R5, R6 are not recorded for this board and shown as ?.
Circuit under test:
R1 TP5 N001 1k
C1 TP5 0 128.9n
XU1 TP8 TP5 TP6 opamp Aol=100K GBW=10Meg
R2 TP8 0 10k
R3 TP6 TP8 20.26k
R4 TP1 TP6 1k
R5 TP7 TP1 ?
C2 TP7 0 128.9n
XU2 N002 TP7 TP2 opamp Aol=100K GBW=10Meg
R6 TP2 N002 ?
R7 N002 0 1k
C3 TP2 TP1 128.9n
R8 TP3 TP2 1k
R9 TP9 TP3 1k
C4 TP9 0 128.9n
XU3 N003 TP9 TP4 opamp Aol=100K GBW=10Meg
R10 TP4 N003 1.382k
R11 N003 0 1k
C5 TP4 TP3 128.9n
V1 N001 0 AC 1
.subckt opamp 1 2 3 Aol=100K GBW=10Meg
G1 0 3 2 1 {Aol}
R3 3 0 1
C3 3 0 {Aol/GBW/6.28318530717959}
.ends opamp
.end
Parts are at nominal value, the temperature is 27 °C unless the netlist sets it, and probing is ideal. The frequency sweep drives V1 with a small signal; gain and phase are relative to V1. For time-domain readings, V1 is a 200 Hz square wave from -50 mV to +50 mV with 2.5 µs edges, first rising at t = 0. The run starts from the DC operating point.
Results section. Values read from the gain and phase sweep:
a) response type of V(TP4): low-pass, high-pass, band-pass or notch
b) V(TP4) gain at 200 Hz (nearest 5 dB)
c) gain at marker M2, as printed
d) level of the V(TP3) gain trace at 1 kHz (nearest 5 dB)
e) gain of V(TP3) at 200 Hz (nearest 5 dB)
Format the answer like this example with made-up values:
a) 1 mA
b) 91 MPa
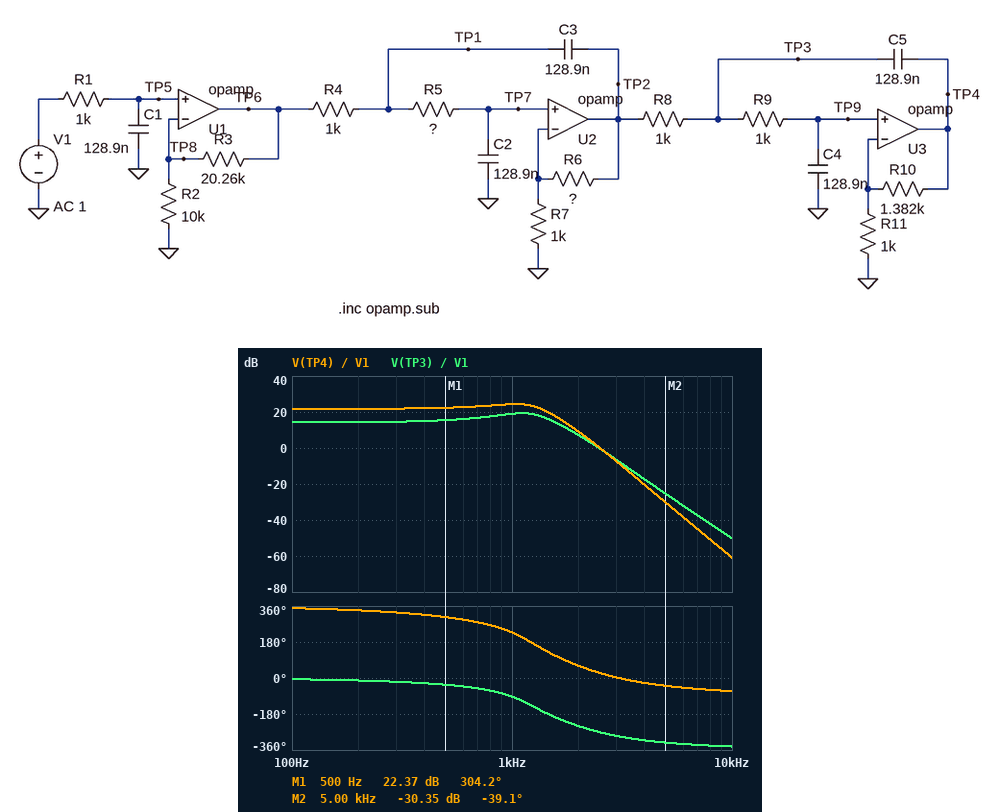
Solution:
a) low-pass
b) 20 dB
c) -30.35 dB
d) 20 dB
e) 15 dB
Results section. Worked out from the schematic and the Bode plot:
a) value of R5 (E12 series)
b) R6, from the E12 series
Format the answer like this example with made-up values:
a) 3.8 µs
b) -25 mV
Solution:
a) 390 Ω
b) 680 Ω
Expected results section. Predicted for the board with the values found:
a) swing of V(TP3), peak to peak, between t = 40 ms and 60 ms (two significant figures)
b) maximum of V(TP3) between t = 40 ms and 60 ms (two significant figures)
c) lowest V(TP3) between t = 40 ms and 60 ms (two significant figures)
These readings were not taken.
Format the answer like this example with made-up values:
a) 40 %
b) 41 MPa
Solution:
a) 940 mV
b) 470 mV
c) -470 mV
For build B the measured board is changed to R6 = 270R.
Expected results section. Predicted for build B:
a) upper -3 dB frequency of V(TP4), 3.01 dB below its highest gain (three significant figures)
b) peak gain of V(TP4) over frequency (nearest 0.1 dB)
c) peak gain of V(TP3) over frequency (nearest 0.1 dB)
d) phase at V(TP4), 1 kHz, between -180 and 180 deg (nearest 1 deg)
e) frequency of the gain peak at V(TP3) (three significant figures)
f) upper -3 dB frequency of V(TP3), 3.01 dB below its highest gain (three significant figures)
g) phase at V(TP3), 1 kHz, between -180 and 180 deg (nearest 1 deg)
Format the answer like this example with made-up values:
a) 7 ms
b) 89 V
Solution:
a) 1.31 kHz
b) 20.0 dB
c) 14.7 dB
d) -145 deg
e) 1.05 kHz
f) 1.38 kHz
g) -106 deg
